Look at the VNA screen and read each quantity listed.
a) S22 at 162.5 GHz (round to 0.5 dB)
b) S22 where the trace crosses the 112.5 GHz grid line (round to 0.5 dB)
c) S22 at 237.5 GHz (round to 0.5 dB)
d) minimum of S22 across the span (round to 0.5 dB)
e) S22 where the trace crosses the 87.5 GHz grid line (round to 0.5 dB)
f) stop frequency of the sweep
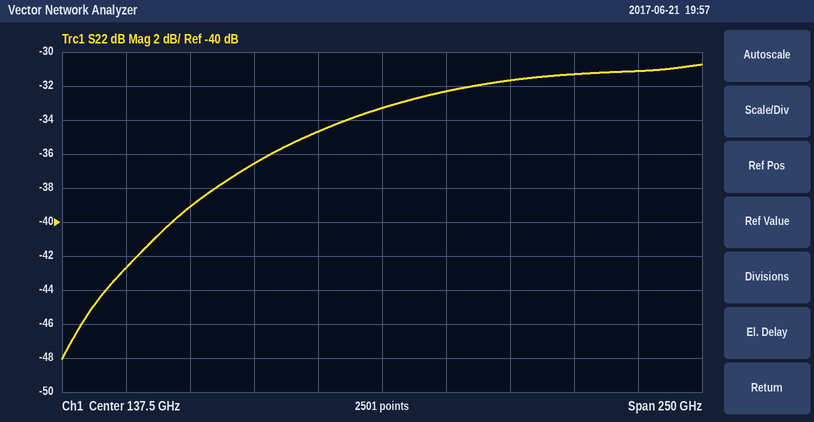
-32.5 dB
-34.5 dB
-31.0 dB
-48.0 dB
-36.5 dB
262.5 GHz
